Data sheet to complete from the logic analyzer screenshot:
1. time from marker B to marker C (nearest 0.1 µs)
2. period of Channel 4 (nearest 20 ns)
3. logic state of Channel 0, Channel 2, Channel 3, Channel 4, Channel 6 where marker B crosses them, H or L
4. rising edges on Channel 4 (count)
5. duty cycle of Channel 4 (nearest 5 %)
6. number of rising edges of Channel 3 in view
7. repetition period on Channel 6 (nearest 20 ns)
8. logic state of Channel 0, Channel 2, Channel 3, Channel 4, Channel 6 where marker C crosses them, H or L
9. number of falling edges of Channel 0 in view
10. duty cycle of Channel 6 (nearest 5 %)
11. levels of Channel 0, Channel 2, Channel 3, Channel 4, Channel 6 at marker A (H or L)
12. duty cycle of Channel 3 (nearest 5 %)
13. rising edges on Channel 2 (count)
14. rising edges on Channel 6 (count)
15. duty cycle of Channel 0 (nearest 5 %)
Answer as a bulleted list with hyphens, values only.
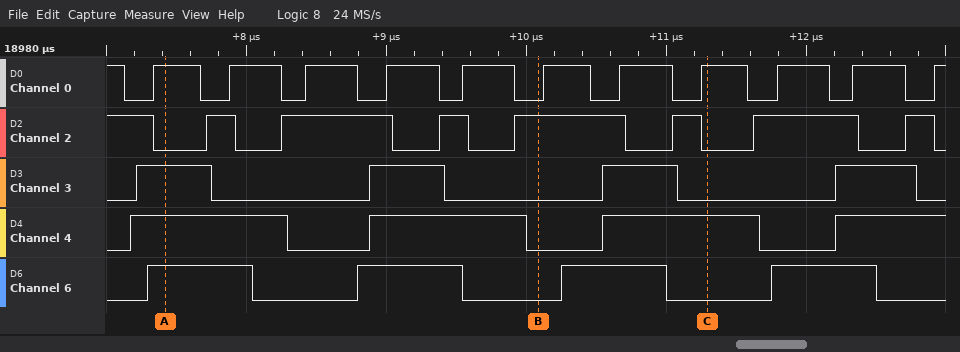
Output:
- 1.2 µs
- 1680 ns
- Channel 0=L, Channel 2=H, Channel 3=L, Channel 4=L, Channel 6=L
- 4
- 65 %
- 4
- 1480 ns
- Channel 0=H, Channel 2=L, Channel 3=L, Channel 4=H, Channel 6=L
- 11
- 50 %
- Channel 0=H, Channel 2=L, Channel 3=H, Channel 4=H, Channel 6=H
- 35 %
- 7
- 4
- 65 %
